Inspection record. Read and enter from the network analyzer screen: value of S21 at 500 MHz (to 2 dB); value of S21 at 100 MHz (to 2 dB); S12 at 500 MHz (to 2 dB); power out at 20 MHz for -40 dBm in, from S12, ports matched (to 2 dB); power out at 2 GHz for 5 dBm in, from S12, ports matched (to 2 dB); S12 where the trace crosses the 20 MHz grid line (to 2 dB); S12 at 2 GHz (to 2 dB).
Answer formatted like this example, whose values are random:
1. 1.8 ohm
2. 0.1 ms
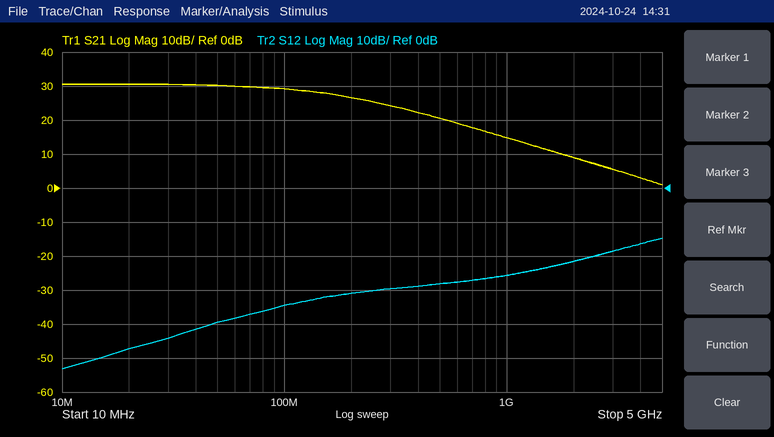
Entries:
1. 20 dB
2. 30 dB
3. -28 dB
4. -88 dBm
5. -16 dBm
6. -48 dB
7. -22 dB
